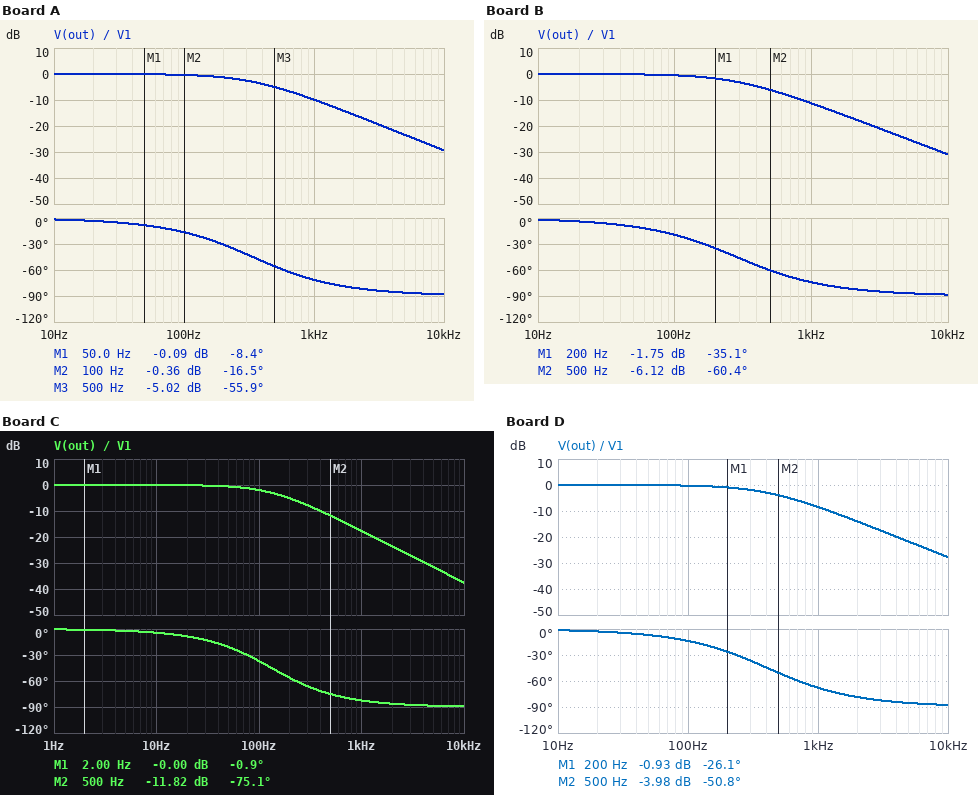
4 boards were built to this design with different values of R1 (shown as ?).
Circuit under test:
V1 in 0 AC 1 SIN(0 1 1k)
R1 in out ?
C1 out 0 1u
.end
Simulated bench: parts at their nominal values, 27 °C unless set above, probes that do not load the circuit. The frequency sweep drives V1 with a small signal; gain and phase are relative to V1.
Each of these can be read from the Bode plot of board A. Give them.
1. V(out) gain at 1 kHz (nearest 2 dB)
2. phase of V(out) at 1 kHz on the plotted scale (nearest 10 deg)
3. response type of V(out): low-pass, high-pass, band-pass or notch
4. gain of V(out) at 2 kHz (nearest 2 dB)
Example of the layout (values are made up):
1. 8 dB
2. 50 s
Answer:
1. -10 dB
2. -70 deg
3. low-pass
4. -16 dB
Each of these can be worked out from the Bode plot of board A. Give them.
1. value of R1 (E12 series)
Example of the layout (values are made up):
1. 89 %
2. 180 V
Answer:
1. 470 Ω
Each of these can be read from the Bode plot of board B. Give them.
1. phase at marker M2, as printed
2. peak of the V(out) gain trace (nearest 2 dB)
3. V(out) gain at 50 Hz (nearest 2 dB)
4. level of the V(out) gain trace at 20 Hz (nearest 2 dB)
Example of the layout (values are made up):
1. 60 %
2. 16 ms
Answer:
1. -60.4 deg
2. 0 dB
3. 0 dB
4. 0 dB
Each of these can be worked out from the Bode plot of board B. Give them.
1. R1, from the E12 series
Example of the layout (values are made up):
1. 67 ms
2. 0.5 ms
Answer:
1. 560 Ω
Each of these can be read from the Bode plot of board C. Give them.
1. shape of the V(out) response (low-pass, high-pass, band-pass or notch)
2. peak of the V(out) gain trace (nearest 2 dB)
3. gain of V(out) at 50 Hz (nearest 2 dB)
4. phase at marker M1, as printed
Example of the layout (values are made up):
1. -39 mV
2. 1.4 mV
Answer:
1. low-pass
2. 0 dB
3. 0 dB
4. -0.9 deg
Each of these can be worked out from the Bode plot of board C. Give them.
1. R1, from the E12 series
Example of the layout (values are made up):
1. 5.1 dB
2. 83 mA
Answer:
1. 1.2 kΩ
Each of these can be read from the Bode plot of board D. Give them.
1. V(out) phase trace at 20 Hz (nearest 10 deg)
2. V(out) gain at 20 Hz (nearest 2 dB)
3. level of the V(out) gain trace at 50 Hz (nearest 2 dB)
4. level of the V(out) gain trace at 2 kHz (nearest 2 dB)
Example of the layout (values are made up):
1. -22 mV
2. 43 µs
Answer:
1. 0 deg
2. 0 dB
3. 0 dB
4. -14 dB
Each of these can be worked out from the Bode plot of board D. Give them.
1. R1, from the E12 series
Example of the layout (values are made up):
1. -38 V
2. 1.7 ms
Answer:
1. 390 Ω
